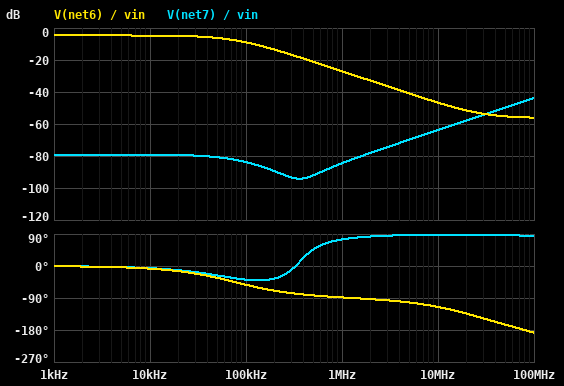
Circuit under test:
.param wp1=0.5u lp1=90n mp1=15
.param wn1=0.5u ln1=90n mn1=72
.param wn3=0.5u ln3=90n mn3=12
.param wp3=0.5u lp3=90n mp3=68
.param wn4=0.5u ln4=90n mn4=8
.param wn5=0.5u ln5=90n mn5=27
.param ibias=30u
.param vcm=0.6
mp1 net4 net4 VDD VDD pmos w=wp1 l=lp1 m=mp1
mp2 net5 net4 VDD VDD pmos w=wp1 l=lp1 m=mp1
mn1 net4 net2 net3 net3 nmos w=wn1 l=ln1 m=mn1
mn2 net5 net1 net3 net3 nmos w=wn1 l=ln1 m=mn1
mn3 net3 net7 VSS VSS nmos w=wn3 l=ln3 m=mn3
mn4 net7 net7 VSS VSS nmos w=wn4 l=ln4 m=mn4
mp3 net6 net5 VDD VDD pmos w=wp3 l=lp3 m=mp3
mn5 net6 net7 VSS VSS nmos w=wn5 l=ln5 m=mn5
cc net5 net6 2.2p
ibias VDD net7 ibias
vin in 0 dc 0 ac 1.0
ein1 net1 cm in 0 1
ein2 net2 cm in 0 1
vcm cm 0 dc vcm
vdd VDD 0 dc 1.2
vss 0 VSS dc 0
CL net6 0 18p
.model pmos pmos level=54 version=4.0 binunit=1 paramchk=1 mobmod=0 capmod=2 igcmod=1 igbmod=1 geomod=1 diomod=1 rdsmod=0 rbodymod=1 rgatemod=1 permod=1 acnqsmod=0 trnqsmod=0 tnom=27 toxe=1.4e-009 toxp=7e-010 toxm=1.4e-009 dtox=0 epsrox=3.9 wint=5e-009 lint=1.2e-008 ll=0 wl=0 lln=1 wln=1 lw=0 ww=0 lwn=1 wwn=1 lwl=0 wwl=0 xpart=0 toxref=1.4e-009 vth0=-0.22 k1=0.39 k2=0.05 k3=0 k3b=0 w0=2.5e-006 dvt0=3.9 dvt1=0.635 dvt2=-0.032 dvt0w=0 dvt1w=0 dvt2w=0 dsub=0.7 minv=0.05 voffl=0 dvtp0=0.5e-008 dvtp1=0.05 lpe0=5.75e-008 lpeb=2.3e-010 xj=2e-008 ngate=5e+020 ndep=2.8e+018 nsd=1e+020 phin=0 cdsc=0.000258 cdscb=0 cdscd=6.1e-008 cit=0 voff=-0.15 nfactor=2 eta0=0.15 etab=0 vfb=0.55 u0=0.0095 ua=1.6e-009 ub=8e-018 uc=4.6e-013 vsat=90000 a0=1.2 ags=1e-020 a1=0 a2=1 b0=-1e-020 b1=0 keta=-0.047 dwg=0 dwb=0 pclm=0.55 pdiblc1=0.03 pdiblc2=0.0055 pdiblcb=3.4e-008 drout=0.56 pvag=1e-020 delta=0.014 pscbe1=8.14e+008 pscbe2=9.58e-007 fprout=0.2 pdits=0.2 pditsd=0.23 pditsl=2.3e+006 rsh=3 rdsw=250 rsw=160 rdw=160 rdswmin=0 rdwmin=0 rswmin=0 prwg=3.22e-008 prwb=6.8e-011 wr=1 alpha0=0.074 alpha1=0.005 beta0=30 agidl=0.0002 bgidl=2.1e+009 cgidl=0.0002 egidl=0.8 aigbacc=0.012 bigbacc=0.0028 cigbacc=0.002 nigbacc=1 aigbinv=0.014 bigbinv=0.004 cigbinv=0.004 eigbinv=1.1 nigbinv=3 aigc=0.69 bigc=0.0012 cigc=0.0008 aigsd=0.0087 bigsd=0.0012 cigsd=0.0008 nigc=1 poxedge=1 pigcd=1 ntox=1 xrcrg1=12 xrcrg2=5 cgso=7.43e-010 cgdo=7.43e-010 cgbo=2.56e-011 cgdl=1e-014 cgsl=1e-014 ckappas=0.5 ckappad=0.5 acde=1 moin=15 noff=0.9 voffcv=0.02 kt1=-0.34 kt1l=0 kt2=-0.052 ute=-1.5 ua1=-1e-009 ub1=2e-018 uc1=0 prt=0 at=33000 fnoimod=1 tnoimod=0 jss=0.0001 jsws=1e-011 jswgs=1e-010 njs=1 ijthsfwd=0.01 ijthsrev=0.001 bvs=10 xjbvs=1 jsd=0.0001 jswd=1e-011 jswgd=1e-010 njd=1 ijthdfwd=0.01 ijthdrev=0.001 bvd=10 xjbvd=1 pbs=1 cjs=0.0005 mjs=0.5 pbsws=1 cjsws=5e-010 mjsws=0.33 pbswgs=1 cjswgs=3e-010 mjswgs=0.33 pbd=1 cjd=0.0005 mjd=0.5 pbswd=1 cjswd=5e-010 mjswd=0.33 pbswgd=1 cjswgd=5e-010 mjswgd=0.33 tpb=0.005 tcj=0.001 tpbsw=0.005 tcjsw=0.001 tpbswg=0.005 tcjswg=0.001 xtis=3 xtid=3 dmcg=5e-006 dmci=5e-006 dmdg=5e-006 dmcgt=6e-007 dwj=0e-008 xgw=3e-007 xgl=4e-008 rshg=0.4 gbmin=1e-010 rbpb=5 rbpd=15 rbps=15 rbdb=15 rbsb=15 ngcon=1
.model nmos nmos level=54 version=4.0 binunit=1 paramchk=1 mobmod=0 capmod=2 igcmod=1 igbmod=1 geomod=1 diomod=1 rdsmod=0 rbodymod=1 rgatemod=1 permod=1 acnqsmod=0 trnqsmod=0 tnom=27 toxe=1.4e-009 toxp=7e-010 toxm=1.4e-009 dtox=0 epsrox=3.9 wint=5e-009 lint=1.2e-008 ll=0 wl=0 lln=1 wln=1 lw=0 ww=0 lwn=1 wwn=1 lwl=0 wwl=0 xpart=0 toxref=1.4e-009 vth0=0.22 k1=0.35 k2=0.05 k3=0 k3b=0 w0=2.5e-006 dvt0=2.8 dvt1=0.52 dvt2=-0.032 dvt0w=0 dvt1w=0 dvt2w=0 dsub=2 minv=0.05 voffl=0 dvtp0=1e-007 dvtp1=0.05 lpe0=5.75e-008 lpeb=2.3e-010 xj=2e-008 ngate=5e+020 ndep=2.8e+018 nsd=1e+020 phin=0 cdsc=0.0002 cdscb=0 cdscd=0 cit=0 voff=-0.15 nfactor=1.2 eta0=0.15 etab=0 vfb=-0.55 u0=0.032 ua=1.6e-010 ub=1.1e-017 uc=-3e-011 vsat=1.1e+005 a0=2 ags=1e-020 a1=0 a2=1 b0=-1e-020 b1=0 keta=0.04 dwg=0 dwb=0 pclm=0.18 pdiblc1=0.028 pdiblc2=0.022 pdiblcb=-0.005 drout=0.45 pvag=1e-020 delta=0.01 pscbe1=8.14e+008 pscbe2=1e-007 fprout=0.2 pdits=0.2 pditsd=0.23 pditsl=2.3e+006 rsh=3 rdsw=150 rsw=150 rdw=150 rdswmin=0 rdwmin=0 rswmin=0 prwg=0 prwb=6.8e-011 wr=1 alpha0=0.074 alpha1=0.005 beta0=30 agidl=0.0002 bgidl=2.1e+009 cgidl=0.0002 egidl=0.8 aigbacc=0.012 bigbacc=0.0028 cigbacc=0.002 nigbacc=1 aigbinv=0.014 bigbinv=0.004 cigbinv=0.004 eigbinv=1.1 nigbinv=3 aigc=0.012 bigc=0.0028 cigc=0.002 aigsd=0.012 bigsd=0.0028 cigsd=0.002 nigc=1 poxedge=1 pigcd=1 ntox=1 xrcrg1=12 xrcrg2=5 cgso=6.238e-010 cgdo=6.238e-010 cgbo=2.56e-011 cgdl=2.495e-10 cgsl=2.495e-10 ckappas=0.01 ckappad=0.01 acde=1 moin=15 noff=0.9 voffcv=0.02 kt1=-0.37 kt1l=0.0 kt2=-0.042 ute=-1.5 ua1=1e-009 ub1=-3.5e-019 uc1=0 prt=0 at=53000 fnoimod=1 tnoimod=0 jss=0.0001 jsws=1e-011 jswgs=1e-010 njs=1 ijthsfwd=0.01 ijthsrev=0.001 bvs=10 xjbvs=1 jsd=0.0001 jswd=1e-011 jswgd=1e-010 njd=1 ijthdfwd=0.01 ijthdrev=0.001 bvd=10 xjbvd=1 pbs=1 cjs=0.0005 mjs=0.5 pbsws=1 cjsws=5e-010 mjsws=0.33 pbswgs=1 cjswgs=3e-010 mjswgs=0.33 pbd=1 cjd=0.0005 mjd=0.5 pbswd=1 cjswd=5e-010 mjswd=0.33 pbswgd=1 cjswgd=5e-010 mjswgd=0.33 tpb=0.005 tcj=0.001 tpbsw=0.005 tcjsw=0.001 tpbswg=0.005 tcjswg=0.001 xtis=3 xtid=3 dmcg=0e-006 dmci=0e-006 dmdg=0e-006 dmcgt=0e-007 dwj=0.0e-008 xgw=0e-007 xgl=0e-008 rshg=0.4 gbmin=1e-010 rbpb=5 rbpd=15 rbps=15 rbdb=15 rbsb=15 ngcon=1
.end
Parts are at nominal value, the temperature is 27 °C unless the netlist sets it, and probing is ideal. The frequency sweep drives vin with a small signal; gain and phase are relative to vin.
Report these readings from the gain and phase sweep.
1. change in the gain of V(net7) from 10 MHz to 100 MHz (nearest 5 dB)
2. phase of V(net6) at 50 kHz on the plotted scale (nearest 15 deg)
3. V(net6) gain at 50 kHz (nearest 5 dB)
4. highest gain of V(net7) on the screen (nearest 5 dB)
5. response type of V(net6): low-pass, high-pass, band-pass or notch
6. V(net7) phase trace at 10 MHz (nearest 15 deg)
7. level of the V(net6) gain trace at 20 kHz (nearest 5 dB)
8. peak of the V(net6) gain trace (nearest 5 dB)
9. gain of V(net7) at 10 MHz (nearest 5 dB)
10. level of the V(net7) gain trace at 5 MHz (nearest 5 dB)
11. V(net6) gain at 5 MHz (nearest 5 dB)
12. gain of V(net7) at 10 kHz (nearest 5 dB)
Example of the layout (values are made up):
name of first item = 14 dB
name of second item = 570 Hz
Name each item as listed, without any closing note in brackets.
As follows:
change in the gain of V(net7) from 10 MHz to 100 MHz = 20 dB
phase of V(net6) at 50 kHz on the plotted scale = -30 deg
V(net6) gain at 50 kHz = -5 dB
highest gain of V(net7) on the screen = -45 dB
response type of V(net6): low-pass, high-pass, band-pass or notch = low-pass
V(net7) phase trace at 10 MHz = 90 deg
level of the V(net6) gain trace at 20 kHz = -5 dB
peak of the V(net6) gain trace = -5 dB
gain of V(net7) at 10 MHz = -65 dB
level of the V(net7) gain trace at 5 MHz = -70 dB
V(net6) gain at 5 MHz = -40 dB
gain of V(net7) at 10 kHz = -80 dB
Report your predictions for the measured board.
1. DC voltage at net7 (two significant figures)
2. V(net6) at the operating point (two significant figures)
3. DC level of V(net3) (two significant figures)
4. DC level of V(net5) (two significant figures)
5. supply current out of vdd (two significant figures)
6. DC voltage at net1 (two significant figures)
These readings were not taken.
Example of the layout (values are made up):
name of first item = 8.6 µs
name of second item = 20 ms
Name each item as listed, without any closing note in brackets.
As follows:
DC voltage at net7 = 390 mV
V(net6) at the operating point = 520 mV
DC level of V(net3) = 340 mV
DC level of V(net5) = 820 mV
supply current out of vdd = 180 µA
DC voltage at net1 = 600 mV
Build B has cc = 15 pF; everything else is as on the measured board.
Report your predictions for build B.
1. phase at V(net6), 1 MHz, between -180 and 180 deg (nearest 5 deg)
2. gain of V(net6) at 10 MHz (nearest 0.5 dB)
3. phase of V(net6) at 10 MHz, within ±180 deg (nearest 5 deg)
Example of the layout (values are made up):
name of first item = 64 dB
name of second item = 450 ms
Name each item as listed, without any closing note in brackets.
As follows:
phase at V(net6), 1 MHz, between -180 and 180 deg = -95 deg
gain of V(net6) at 10 MHz = -58.0 dB
phase of V(net6) at 10 MHz, within ±180 deg = -135 deg
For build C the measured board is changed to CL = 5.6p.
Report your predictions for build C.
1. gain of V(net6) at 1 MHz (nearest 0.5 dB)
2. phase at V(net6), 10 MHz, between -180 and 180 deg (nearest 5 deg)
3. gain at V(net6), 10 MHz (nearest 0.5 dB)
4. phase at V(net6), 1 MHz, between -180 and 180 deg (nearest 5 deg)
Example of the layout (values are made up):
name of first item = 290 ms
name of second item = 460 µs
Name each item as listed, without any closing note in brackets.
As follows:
gain of V(net6) at 1 MHz = -26.5 dB
phase at V(net6), 10 MHz, between -180 and 180 deg = -95 deg
gain at V(net6), 10 MHz = -45.0 dB
phase at V(net6), 1 MHz, between -180 and 180 deg = -85 deg
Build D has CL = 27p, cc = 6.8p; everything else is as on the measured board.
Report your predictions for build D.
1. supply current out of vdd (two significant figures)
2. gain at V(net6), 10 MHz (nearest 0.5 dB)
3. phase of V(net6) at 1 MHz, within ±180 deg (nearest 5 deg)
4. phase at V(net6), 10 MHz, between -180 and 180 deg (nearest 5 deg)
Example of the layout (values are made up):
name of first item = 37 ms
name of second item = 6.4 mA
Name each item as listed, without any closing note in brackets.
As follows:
supply current out of vdd = 180 µA
gain at V(net6), 10 MHz = -55.5 dB
phase of V(net6) at 1 MHz, within ±180 deg = -95 deg
phase at V(net6), 10 MHz, between -180 and 180 deg = -135 deg
